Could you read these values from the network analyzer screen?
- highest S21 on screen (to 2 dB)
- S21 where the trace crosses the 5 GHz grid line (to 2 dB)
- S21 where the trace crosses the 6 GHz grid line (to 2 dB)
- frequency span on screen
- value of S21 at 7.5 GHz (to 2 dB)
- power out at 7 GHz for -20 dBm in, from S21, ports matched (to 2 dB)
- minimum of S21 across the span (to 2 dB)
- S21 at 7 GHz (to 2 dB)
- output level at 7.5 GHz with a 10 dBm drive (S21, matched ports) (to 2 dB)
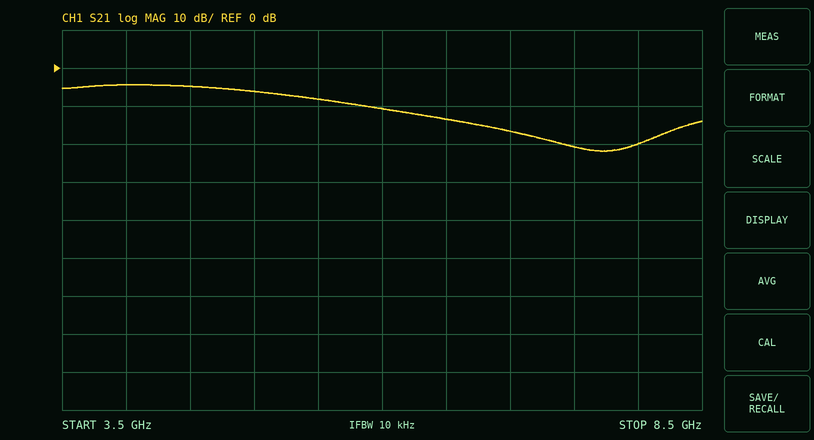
-4 dB
-6 dB
-10 dB
5 GHz
-20 dB
-36 dBm
-22 dB
-16 dB
-10 dBm
